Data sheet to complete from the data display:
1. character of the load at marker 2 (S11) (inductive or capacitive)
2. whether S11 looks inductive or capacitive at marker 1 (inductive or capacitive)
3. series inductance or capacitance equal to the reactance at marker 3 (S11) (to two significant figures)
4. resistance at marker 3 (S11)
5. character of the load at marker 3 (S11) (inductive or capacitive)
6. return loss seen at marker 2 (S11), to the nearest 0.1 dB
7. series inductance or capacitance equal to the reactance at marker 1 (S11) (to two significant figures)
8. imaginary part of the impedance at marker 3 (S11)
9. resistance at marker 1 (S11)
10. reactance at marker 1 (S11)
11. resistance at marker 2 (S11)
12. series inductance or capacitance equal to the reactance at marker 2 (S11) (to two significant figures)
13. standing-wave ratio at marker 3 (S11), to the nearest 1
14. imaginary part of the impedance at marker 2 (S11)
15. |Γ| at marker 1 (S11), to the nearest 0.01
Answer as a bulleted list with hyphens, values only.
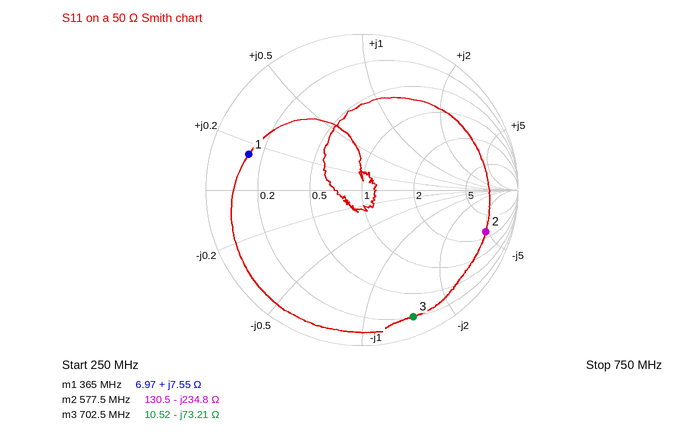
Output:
- capacitive
- inductive
- 3.1 pF
- 10.52 Ω
- capacitive
- 1.5 dB
- 3.3 nH
- -73.21 Ω
- 6.97 Ω
- +7.55 Ω
- 130.5 Ω
- 1.2 pF
- 15
- -234.8 Ω
- 0.76
